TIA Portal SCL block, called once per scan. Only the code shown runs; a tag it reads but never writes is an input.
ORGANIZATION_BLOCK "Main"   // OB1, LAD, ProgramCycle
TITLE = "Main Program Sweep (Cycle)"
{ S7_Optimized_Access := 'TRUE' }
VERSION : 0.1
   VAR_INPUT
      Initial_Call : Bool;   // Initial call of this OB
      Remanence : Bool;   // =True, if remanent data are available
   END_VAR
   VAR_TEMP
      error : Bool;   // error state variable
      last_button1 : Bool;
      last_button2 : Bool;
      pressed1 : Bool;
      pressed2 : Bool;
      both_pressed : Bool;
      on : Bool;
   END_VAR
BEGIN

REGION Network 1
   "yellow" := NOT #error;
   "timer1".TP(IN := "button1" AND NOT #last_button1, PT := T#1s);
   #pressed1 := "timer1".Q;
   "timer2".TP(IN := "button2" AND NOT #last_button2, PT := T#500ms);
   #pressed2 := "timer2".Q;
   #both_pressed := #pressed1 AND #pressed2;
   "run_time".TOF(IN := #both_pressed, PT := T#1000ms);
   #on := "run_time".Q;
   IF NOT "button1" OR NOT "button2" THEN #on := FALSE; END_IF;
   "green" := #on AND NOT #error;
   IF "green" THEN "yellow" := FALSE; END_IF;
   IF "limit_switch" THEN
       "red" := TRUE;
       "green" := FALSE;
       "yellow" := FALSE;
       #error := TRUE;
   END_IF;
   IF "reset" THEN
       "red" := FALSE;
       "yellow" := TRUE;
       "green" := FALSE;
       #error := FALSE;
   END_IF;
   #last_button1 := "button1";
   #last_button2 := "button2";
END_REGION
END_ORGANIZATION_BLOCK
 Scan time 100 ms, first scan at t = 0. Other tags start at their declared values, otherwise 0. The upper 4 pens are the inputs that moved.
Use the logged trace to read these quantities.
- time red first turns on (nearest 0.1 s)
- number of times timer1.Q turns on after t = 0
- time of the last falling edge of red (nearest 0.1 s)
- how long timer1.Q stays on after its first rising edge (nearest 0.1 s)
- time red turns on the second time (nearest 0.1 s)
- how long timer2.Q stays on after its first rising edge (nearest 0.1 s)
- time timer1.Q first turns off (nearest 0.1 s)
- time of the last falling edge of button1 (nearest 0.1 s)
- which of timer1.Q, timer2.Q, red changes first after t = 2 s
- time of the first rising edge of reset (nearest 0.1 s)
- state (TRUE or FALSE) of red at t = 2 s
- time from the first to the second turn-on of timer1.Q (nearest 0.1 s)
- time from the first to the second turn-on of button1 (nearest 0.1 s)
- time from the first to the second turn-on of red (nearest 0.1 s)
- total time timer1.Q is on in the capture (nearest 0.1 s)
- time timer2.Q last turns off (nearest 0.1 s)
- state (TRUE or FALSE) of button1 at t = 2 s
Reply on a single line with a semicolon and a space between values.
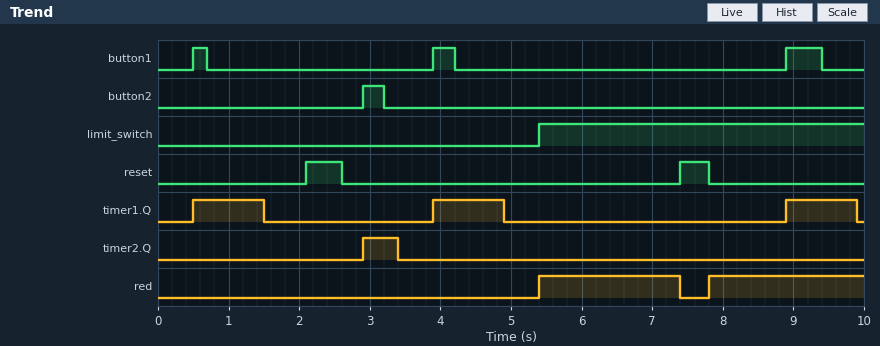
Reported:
5.4 s; 3; 7.4 s; 1.0 s; 7.8 s; 0.5 s; 1.5 s; 9.4 s; timer2.Q; 2.1 s; FALSE; 3.4 s; 3.4 s; 2.4 s; 3.0 s; 3.4 s; FALSE
